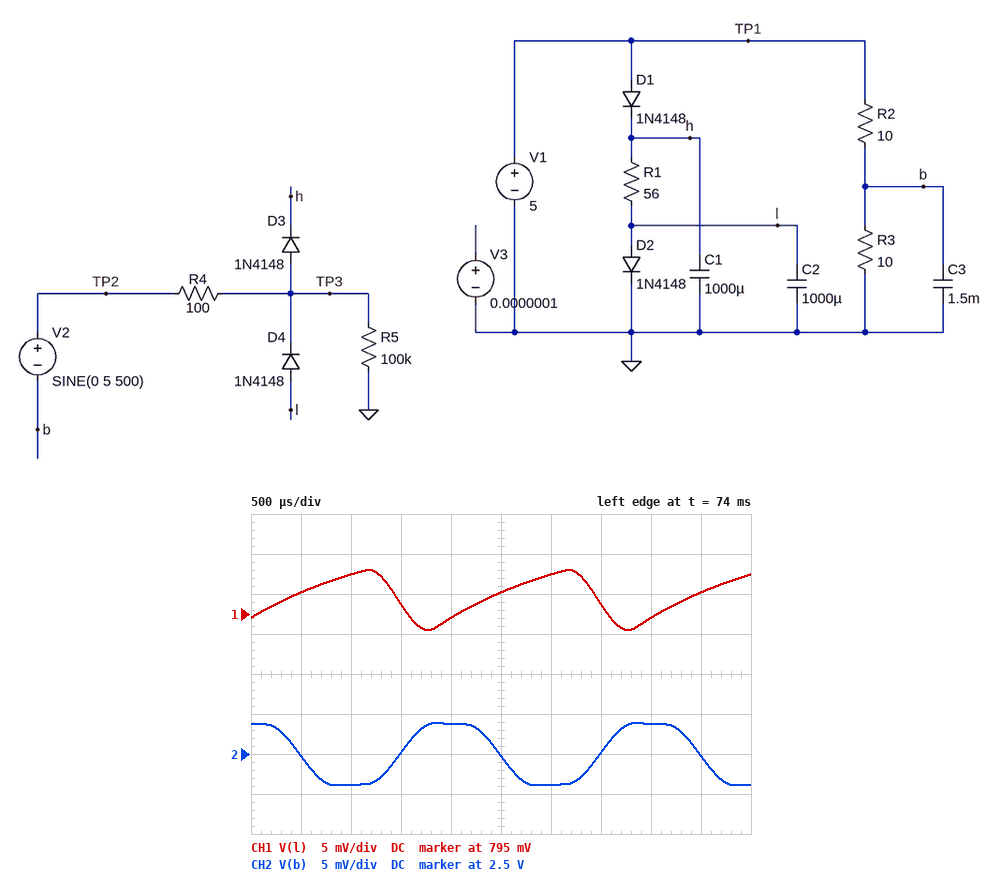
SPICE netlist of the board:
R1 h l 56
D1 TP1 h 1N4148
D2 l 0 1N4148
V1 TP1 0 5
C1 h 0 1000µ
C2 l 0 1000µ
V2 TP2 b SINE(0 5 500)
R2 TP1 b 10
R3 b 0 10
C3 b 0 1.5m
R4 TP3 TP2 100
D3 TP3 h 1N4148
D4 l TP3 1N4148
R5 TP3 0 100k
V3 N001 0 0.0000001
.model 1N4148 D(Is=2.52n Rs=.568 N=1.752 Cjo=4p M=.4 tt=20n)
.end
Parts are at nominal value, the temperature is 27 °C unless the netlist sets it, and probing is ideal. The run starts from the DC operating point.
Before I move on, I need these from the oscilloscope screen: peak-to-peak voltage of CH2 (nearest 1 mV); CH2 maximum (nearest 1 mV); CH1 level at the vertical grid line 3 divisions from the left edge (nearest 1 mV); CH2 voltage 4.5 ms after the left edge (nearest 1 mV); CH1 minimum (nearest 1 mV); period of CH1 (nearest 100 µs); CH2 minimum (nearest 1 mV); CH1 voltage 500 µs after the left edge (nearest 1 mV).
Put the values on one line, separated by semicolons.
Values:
8 mV; 2.504 V; 796 mV; 2.500 V; 793 mV; 2.0 ms; 2.496 V; 798 mV
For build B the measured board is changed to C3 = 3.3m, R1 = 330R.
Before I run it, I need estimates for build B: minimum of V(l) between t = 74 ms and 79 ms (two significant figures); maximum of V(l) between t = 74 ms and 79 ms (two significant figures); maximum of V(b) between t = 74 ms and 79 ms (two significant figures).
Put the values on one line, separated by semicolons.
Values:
660 mV; 670 mV; 2.5 V
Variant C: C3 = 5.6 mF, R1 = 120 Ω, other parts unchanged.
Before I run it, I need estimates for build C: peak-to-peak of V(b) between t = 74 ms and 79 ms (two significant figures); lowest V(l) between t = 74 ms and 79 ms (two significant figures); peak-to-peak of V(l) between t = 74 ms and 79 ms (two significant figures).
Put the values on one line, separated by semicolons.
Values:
2.0 mV; 740 mV; 7.5 mV
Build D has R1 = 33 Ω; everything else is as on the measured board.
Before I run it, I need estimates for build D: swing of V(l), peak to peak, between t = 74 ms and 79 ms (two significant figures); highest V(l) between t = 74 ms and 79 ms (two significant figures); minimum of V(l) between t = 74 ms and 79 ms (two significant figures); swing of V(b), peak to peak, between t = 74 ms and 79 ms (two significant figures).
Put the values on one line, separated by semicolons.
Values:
7.5 mV; 850 mV; 840 mV; 8.0 mV
